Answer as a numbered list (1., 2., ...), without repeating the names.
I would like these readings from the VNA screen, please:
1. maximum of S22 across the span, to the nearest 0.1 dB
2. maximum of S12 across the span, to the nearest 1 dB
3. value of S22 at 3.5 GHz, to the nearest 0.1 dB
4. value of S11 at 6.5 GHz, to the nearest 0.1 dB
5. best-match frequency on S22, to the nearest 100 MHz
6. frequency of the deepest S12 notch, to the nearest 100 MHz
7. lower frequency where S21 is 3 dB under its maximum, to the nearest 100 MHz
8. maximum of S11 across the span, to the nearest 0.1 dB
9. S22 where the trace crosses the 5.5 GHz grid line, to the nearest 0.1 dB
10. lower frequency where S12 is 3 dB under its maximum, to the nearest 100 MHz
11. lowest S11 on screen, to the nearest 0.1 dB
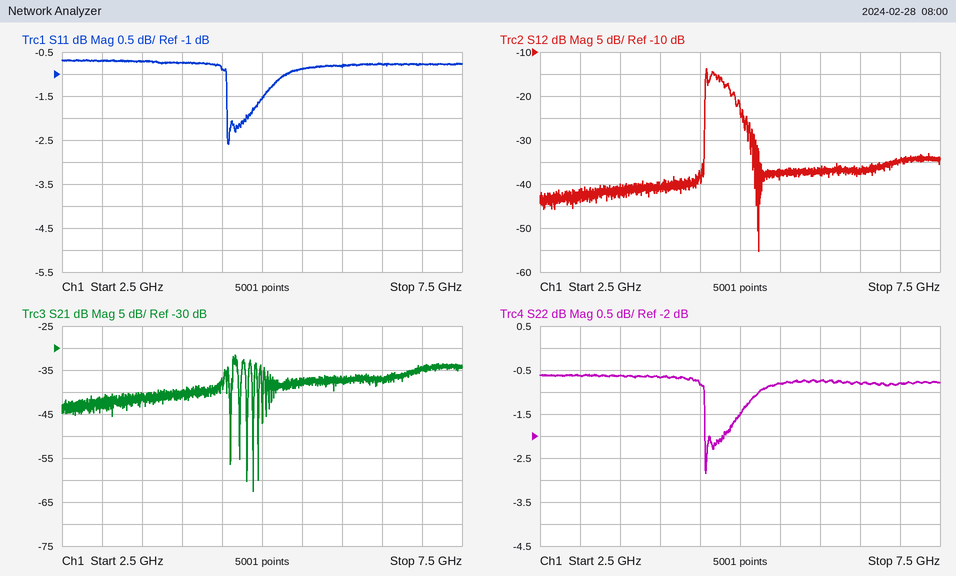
1. -0.6 dB
2. -14 dB
3. -0.6 dB
4. -0.8 dB
5. 4.6 GHz
6. 5.2 GHz
7. 4.6 GHz
8. -0.7 dB
9. -0.8 dB
10. 4.6 GHz
11. -2.6 dB
